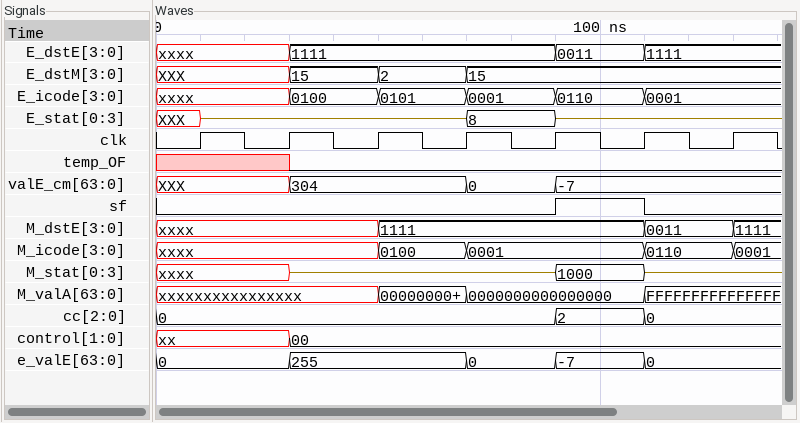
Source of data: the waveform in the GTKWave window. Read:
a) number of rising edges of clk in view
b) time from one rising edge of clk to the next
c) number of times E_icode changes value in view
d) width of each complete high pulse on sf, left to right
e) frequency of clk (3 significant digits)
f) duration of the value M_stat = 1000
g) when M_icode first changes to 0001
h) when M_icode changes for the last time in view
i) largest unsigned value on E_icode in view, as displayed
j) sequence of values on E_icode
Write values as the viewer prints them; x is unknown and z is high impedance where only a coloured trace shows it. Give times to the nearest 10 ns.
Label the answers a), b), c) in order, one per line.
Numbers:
a) 7
b) 20 ns
c) 5
d) 20 ns
e) 50.0 MHz
f) 20 ns
g) 70 ns
h) 130 ns
i) 0110
j) xxxx, 0100, 0101, 0001, 0110, 0001
